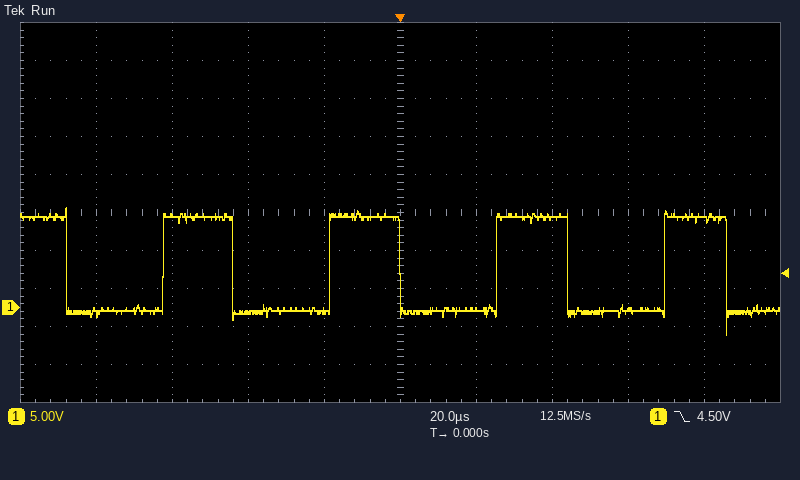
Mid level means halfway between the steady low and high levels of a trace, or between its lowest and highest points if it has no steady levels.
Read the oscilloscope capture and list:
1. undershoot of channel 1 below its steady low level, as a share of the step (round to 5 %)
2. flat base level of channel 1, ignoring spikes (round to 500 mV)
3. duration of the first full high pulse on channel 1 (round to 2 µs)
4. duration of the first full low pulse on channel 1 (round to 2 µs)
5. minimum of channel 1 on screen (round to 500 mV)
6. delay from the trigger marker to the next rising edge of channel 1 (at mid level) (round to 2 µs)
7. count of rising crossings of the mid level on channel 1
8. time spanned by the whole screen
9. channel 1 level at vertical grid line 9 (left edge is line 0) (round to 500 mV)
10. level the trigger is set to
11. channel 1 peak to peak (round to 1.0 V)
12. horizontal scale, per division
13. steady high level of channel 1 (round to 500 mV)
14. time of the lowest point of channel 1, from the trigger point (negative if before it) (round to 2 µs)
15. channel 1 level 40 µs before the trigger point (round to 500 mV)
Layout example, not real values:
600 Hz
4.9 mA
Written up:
25 %
-500 mV
18 µs
26 µs
-3.5 V
26 µs
4
200 µs
11.5 V
4.50 V
17.0 V
20 µs
12.0 V
+86 µs
-500 mV
